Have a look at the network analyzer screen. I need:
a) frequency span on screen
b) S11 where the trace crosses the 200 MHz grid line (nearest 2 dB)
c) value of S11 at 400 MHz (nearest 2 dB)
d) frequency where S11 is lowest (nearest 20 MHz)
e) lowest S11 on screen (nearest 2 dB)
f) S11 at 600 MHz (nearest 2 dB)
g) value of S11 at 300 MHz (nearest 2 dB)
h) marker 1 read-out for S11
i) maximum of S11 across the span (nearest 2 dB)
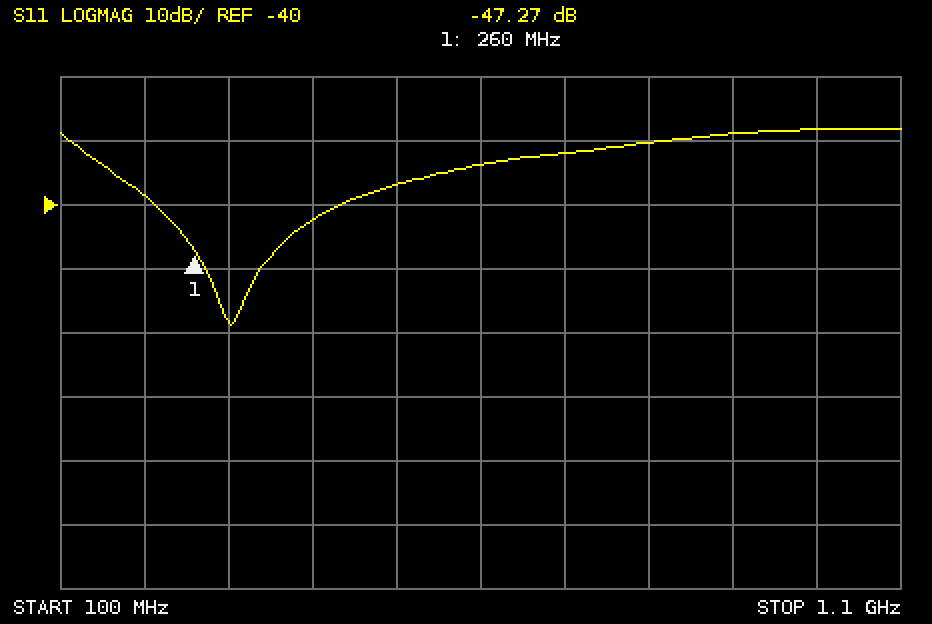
1 GHz
-38 dB
-42 dB
300 MHz
-58 dB
-34 dB
-58 dB
-47.27 dB
-28 dB
